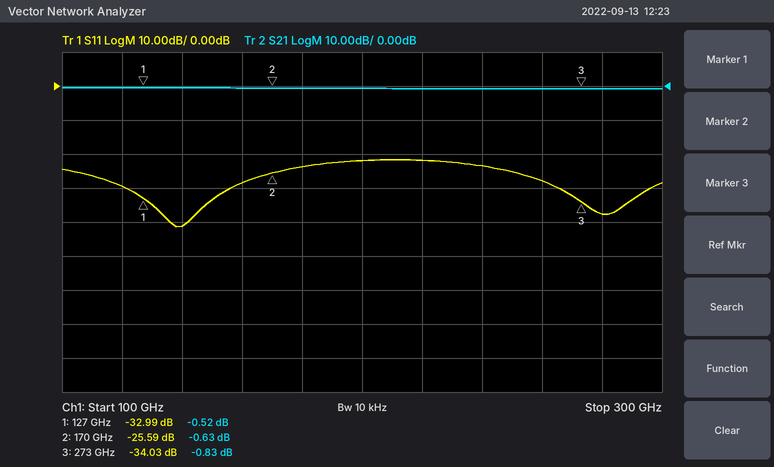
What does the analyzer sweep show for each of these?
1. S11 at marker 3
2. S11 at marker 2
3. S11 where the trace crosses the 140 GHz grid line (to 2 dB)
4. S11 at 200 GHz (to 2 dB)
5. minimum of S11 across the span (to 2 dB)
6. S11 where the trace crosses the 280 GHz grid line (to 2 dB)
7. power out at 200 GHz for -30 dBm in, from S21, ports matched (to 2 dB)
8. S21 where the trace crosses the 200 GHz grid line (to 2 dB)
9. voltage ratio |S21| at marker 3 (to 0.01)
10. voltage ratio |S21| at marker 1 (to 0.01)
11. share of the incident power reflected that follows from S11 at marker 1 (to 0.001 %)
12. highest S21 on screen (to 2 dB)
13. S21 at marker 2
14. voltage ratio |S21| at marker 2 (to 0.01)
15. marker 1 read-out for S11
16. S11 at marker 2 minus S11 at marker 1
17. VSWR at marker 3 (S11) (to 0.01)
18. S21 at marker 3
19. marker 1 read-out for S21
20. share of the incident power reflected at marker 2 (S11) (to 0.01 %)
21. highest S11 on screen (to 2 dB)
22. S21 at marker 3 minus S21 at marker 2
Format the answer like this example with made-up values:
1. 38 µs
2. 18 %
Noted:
1. -34.03 dB
2. -25.59 dB
3. -42 dB
4. -22 dB
5. -42 dB
6. -38 dB
7. -30 dBm
8. 0 dB
9. 0.91
10. 0.94
11. 0.050 %
12. 0 dB
13. -0.63 dB
14. 0.93
15. -32.99 dB
16. 7.40 dB
17. 1.04
18. -0.83 dB
19. -0.52 dB
20. 0.28 %
21. -22 dB
22. -0.20 dB
